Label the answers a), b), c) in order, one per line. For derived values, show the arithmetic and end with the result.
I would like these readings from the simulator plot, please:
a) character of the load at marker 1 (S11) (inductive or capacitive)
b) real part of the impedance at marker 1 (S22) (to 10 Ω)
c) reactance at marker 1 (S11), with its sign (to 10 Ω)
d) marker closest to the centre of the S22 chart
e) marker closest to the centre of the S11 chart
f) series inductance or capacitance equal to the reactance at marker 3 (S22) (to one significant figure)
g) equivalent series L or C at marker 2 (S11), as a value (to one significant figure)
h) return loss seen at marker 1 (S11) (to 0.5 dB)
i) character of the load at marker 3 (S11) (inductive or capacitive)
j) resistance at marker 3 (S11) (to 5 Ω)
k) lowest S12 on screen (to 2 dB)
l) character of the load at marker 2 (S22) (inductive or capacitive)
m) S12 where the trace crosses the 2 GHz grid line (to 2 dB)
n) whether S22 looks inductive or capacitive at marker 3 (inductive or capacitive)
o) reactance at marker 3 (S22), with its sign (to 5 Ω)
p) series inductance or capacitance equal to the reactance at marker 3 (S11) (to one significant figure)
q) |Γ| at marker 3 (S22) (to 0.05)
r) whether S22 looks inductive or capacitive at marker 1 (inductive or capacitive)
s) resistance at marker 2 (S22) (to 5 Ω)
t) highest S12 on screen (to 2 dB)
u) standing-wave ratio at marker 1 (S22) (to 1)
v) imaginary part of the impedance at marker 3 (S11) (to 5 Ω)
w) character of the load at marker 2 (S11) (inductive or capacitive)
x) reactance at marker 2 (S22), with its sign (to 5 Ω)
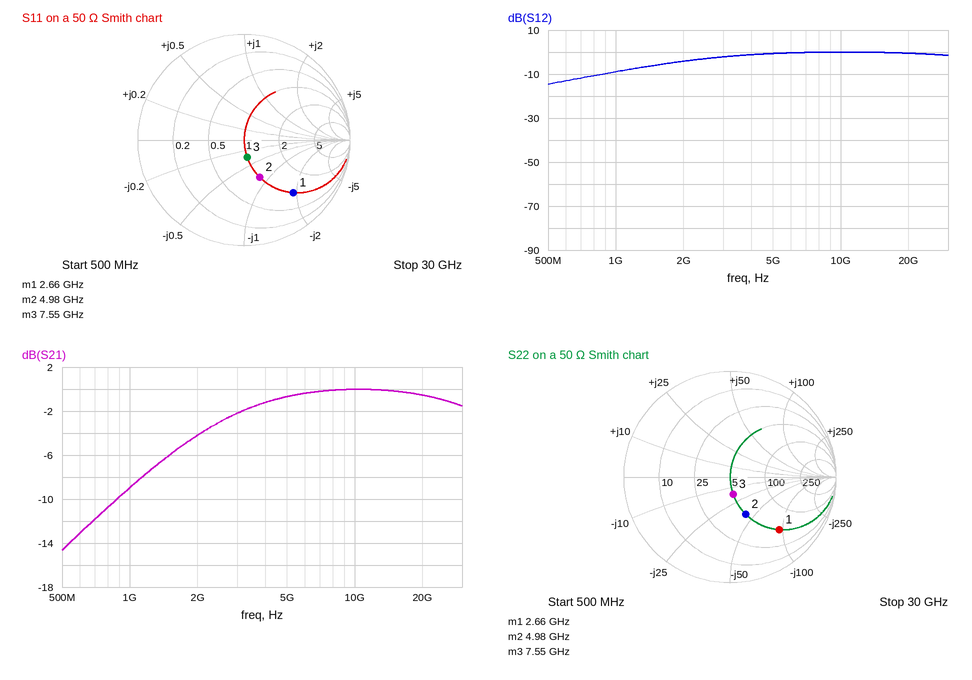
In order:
a) capacitive
b) 50 Ω
c) -90 Ω
d) marker 3
e) marker 3
f) C = 1/(2π × 7.55 GHz × 15 Ω) ≈ 1 pF
g) C = 1/(2π × 4.98 GHz × 40 Ω) ≈ 799 fF, so 800 fF to one significant figure
h) 3.5 dB
i) capacitive
j) 50 Ω
k) -14 dB
l) capacitive
m) -4 dB
n) capacitive
o) -15 Ω
p) C = 1/(2π × 7.55 GHz × 15 Ω) ≈ 1 pF
q) 0.15
r) capacitive
s) 50 Ω
t) 0 dB
u) 5
v) -15 Ω
w) capacitive
x) -40 Ω
